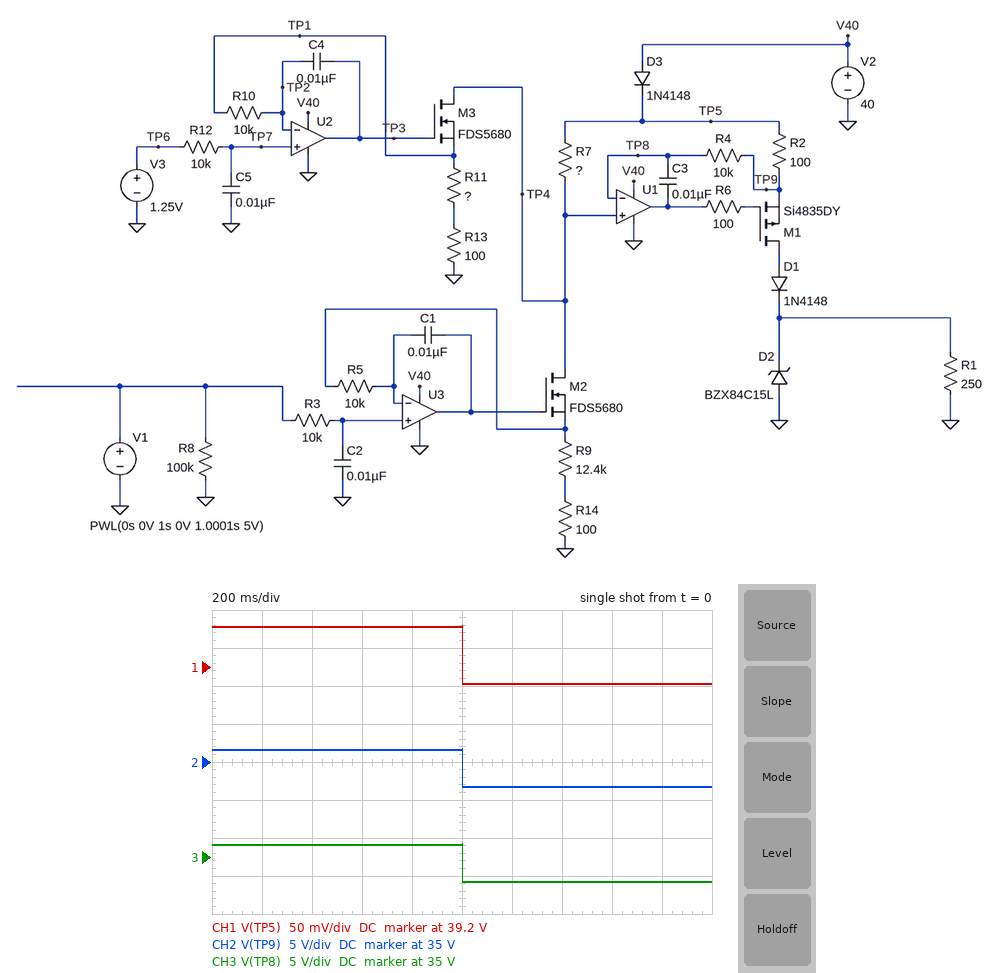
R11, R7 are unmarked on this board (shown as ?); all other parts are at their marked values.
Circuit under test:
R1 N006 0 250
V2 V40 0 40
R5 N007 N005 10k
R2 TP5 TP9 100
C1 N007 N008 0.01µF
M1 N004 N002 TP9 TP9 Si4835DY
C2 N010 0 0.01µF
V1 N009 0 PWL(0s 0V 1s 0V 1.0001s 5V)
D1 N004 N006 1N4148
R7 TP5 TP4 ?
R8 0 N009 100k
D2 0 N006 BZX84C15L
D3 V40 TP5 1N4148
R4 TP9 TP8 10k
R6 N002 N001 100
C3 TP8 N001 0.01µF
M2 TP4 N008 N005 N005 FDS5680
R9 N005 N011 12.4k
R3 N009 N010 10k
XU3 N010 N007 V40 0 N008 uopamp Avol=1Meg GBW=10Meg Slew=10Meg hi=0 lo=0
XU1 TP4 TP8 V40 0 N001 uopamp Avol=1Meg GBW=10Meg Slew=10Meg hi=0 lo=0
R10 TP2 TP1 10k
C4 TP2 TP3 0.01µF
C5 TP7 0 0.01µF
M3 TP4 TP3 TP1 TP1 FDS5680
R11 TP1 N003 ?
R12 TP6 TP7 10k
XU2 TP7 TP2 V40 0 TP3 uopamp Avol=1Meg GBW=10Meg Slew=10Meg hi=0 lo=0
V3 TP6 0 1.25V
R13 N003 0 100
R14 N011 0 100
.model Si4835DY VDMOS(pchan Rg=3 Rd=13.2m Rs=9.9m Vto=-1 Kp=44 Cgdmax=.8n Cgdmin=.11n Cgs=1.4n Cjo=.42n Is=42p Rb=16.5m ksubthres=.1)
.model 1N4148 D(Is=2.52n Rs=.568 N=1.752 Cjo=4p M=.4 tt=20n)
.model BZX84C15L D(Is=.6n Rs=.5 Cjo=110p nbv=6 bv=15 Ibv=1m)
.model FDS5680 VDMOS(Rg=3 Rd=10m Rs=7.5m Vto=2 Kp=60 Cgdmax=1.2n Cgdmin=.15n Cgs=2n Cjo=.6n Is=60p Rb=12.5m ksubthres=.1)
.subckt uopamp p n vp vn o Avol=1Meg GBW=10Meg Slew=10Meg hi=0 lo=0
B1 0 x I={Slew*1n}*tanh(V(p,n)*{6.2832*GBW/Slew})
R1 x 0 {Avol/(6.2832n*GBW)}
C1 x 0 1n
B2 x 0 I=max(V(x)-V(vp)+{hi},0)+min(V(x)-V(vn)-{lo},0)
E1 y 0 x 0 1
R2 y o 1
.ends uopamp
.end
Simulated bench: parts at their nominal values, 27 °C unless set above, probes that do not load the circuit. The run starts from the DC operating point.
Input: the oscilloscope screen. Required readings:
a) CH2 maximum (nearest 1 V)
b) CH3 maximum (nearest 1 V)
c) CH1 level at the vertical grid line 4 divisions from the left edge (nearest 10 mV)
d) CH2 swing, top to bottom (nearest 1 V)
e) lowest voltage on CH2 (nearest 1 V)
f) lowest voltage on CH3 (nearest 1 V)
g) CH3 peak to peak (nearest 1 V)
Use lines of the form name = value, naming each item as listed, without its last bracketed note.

CH2 maximum = 37 V
CH3 maximum = 37 V
CH1 level at the vertical grid line 4 divisions from the left edge = 39.25 V
CH2 swing, top to bottom = 5 V
lowest voltage on CH2 = 32 V
lowest voltage on CH3 = 32 V
CH3 peak to peak = 5 V
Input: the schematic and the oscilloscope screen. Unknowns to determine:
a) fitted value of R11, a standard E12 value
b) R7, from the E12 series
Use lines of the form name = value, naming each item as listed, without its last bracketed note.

fitted value of R11, a standard E12 value = 5.6 kΩ
R7, from the E12 series = 12 kΩ
